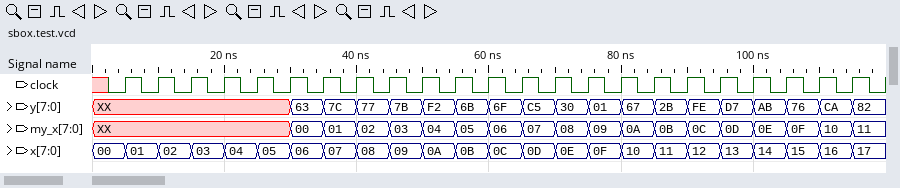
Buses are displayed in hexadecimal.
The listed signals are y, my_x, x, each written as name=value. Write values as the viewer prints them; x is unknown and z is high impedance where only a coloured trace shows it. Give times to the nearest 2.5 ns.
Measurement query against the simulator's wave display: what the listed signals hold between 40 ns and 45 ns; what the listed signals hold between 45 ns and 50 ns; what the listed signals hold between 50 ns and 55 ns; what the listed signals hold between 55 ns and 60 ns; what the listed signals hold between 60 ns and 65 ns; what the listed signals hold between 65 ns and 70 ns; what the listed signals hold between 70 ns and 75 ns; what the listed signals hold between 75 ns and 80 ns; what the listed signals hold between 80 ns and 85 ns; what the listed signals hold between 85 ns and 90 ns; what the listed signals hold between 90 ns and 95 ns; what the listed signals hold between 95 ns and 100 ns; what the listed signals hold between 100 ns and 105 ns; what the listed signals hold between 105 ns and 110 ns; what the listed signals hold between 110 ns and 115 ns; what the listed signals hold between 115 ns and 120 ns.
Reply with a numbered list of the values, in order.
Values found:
1. y=77, my_x=02, x=08
2. y=7B, my_x=03, x=09
3. y=F2, my_x=04, x=0A
4. y=6B, my_x=05, x=0B
5. y=6F, my_x=06, x=0C
6. y=C5, my_x=07, x=0D
7. y=30, my_x=08, x=0E
8. y=01, my_x=09, x=0F
9. y=67, my_x=0A, x=10
10. y=2B, my_x=0B, x=11
11. y=FE, my_x=0C, x=12
12. y=D7, my_x=0D, x=13
13. y=AB, my_x=0E, x=14
14. y=76, my_x=0F, x=15
15. y=CA, my_x=10, x=16
16. y=82, my_x=11, x=17
